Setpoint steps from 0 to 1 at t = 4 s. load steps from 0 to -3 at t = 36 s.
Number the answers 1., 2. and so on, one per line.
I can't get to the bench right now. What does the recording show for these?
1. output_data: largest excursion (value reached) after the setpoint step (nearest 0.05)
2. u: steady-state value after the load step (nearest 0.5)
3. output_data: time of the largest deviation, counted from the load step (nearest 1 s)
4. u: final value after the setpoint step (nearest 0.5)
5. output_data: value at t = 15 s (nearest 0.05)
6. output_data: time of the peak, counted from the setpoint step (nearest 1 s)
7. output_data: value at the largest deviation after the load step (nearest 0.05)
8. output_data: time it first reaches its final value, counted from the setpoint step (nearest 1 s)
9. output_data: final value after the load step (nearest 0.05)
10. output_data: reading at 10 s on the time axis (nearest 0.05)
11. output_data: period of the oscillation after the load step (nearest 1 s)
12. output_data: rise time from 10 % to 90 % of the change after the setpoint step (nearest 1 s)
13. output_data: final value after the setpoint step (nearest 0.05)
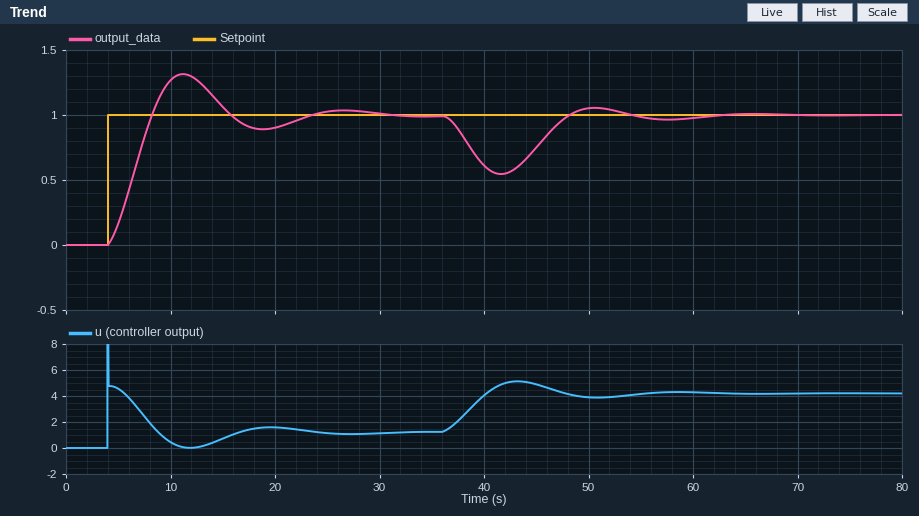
1. 1.30
2. 4.0
3. 6 s
4. 1.0
5. 1.05
6. 7 s
7. 0.55
8. 4 s
9. 1.00
10. 1.25
11. 16 s
12. 3 s
13. 1.00
